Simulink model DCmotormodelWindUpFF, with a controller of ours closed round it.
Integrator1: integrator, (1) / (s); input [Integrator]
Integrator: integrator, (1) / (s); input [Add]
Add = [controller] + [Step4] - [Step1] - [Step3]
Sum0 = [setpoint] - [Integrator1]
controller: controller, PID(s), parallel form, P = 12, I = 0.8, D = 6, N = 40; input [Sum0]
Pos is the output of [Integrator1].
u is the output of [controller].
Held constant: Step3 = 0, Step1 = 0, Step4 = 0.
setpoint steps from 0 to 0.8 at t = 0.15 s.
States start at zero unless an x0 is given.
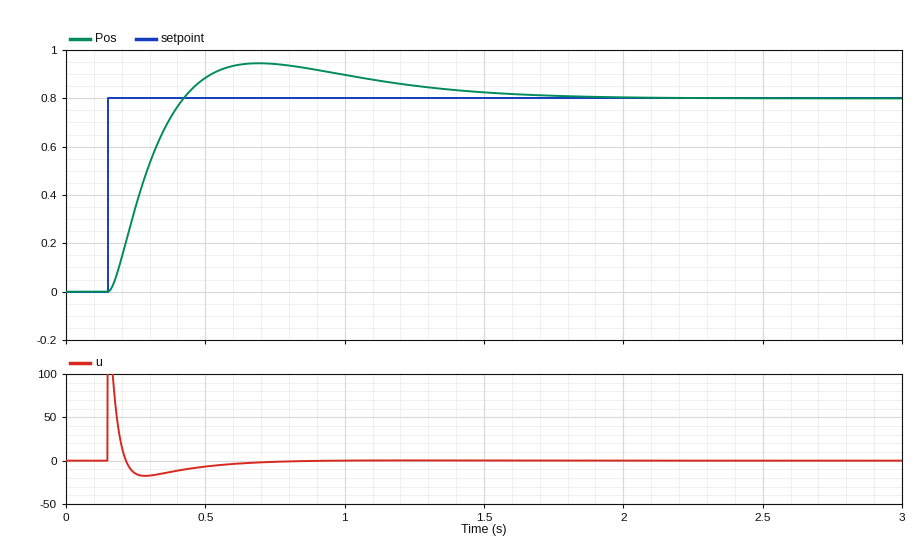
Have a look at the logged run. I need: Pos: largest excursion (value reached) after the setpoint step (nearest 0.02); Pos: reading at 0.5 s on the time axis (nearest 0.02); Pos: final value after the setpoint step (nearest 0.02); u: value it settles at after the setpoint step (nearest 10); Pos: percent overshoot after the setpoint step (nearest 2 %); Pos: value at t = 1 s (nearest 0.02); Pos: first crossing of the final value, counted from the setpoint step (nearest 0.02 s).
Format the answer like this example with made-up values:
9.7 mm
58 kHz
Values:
0.94
0.88
0.80
0
18 %
0.90
0.28 s
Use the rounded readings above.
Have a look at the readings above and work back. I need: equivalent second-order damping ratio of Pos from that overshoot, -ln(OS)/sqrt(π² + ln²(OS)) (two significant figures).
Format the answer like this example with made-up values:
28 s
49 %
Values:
0.48
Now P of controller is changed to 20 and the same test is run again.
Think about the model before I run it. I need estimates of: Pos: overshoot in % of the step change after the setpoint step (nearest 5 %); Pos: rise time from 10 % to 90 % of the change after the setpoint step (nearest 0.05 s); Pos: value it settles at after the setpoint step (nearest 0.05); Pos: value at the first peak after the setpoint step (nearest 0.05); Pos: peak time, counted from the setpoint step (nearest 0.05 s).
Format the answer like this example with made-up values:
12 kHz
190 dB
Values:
25 %
0.15 s
0.80
1.00
0.45 s
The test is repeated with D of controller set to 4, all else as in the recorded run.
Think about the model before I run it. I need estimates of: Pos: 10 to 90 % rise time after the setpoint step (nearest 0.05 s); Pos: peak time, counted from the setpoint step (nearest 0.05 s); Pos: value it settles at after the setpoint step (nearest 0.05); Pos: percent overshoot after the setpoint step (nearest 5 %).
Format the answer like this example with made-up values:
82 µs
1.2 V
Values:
0.25 s
0.65 s
0.80
30 %
